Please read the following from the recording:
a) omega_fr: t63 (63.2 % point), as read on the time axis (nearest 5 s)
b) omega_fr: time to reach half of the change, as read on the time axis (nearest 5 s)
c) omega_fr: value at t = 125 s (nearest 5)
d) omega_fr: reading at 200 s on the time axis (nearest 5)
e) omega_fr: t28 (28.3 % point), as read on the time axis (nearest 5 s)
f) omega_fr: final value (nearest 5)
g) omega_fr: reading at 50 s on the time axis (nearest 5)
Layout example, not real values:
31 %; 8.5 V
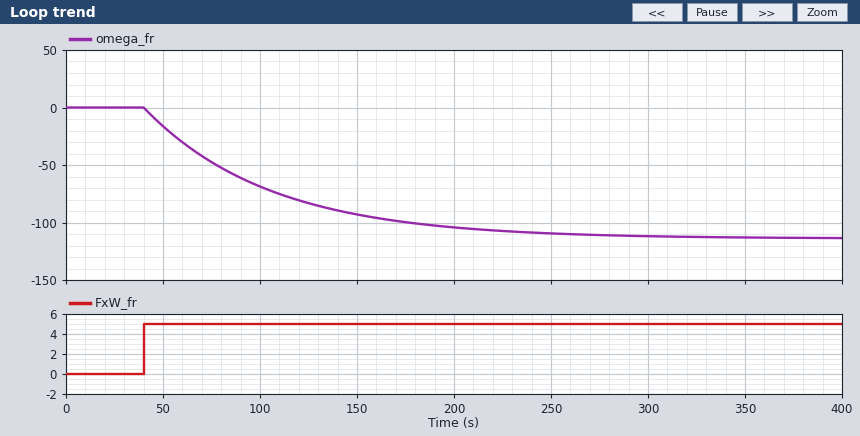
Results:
105 s; 85 s; -85; -105; 60 s; -115; -15
